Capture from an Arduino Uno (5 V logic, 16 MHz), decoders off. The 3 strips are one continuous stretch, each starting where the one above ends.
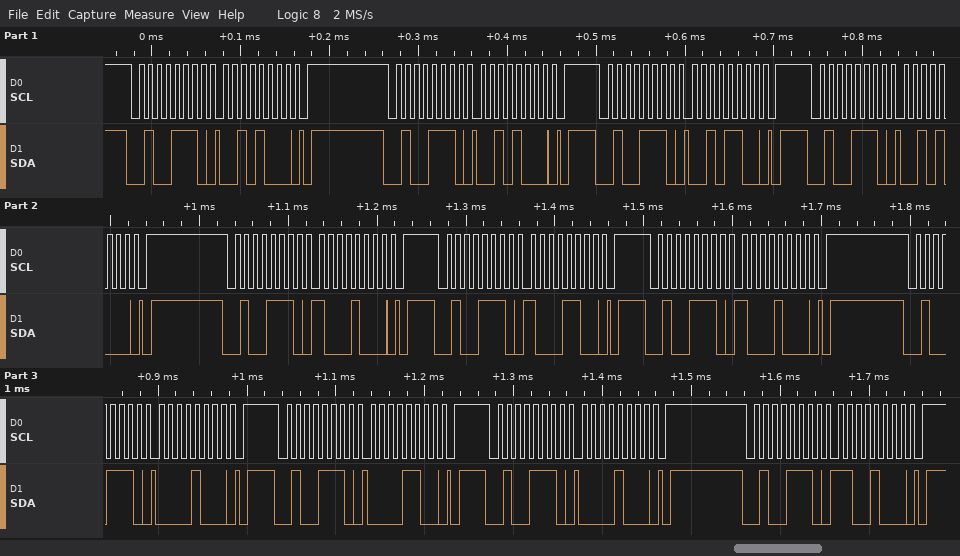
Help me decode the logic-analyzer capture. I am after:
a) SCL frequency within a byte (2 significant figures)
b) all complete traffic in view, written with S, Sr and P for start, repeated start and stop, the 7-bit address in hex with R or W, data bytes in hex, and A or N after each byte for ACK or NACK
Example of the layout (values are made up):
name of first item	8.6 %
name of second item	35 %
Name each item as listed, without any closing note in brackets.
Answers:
SCL frequency within a byte	100 kHz
all complete traffic in view, written with S, Sr and P for start, repeated start and stop, the 7-bit address in hex with R or W, data bytes in hex, and A or N after each byte for ACK or NACK	S 27W A 28 A P S 27W A 28 A P S 27W A 2C A P S 27W A 28 A P S 27W A 88 A P S 27W A 8C A P S 27W A 88 A P S 27W A 08 A P S 27W A 0C A P S 27W A 08 A P S 27W A C8 A P
